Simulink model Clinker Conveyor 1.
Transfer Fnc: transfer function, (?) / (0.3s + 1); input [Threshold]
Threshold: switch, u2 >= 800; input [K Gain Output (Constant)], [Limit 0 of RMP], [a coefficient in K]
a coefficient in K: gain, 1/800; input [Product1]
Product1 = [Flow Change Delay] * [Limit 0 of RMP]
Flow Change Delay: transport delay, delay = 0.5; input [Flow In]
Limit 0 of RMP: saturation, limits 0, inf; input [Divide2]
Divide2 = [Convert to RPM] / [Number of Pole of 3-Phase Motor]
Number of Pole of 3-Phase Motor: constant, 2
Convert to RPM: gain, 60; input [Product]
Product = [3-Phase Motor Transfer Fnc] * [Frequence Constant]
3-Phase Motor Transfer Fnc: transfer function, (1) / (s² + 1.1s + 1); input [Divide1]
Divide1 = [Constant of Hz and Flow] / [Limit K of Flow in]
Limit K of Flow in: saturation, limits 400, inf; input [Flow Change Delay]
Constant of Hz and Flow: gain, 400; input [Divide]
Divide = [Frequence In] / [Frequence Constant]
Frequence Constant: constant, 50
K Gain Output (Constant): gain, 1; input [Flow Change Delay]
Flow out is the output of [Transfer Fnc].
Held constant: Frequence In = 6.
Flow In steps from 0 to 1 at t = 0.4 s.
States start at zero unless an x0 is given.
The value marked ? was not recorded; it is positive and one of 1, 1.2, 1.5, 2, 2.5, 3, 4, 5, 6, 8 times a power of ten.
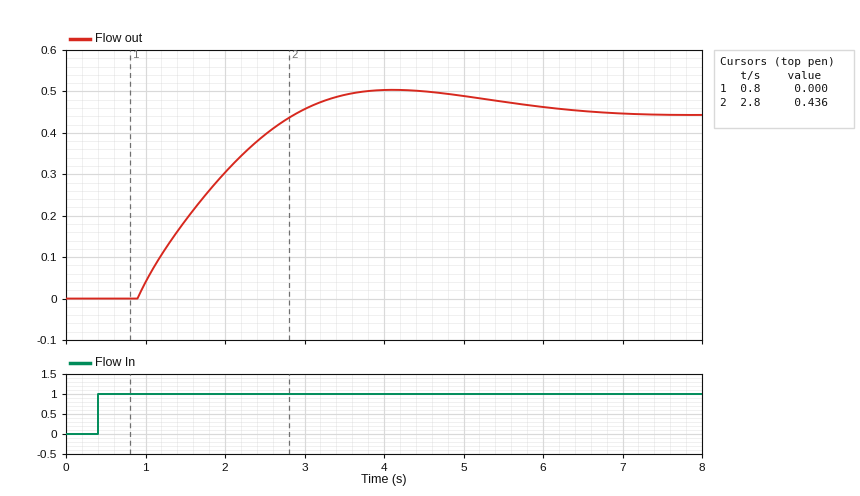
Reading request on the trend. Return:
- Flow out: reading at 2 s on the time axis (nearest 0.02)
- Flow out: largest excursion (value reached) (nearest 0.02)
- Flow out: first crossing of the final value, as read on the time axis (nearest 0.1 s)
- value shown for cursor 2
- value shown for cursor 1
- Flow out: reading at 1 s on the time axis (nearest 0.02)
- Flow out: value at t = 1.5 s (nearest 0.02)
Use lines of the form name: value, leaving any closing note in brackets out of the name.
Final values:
Flow out: reading at 2 s on the time axis: 0.30
Flow out: largest excursion (value reached): 0.50
Flow out: first crossing of the final value, as read on the time axis: 2.9 s
value shown for cursor 2: 0.436
value shown for cursor 1: 0.000
Flow out: reading at 1 s on the time axis: 0.04
Flow out: value at t = 1.5 s: 0.18
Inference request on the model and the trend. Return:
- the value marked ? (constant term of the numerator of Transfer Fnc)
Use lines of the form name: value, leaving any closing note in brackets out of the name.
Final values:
the value marked ?: 2
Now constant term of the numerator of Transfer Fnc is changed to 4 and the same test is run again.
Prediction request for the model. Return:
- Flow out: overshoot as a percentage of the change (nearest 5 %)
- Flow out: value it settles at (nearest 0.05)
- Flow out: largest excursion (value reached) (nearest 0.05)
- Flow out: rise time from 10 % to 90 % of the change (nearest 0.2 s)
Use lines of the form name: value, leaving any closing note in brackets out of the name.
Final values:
Flow out: overshoot as a percentage of the change: 10 %
Flow out: value it settles at: 0.90
Flow out: largest excursion (value reached): 1.00
Flow out: rise time from 10 % to 90 % of the change: 1.6 s
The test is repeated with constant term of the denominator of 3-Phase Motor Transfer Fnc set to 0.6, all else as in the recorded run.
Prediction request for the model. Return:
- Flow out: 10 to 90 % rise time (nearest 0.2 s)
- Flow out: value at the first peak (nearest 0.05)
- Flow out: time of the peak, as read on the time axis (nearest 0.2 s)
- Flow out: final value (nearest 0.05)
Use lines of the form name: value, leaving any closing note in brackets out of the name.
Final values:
Flow out: 10 to 90 % rise time: 2.6 s
Flow out: value at the first peak: 0.80
Flow out: time of the peak, as read on the time axis: 6.2 s
Flow out: final value: 0.75
